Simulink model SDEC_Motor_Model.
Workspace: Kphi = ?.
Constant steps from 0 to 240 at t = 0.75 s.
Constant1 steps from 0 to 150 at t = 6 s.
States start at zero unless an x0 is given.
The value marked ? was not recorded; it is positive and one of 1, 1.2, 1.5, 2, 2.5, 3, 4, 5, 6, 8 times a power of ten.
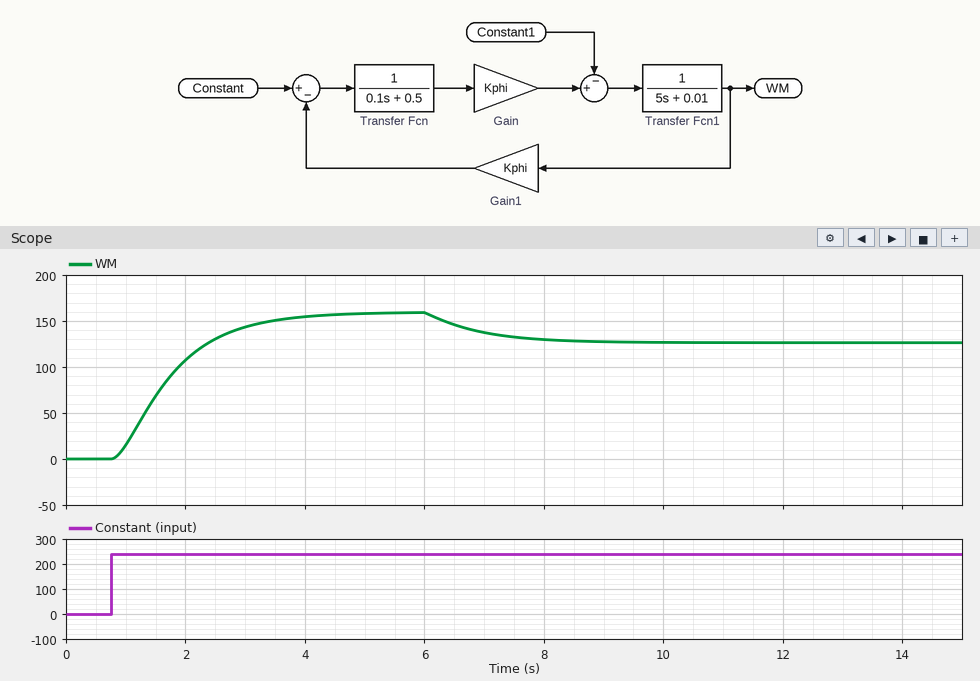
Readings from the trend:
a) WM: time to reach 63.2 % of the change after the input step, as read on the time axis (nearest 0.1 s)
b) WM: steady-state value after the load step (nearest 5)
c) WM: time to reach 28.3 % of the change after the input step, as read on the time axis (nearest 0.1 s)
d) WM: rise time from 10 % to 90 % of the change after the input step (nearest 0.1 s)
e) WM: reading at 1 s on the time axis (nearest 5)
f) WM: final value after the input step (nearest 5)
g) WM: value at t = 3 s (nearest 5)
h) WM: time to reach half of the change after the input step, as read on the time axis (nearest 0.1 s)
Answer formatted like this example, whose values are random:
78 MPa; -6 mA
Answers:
1.9 s; 125; 1.3 s; 2.0 s; 15; 160; 145; 1.6 s
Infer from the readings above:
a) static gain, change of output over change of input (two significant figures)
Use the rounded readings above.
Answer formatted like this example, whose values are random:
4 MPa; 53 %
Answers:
0.67
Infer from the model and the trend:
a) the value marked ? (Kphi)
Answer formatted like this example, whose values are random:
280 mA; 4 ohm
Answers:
1.5
